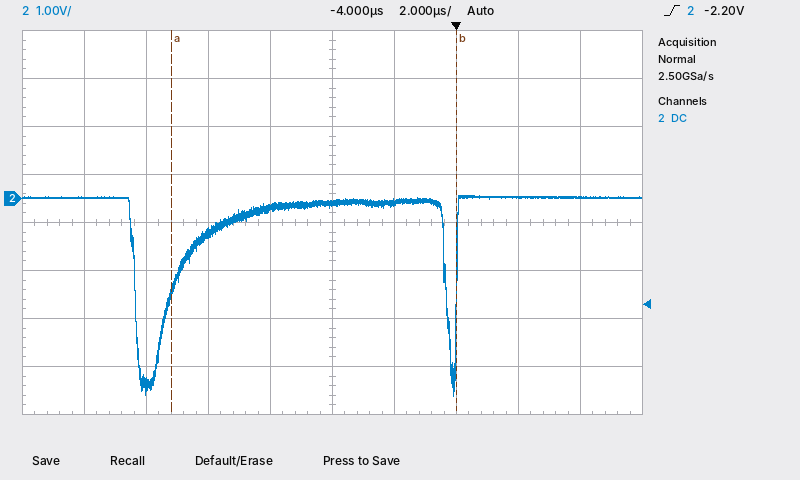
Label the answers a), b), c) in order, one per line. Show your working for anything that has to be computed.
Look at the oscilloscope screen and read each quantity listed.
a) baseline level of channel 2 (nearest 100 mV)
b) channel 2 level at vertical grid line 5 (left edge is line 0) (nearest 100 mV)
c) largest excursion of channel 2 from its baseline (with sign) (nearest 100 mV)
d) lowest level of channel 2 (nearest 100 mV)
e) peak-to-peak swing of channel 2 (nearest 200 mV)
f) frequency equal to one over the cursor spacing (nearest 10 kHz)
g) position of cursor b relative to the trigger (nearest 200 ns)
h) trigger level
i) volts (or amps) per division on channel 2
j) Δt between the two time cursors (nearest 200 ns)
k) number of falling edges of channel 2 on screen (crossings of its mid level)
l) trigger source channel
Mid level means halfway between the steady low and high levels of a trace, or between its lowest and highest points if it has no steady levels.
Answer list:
a) 0.0 V
b) -100 mV
c) -4.1 V − (0.0 V) = -4.1 V
d) -4.1 V
e) 4.2 V
f) 1 / 9.2 µs ≈ 110 kHz
g) 0.0 µs
h) -2.20 V
i) 1 V
j) 9.2 µs
k) 2
l) channel 2
